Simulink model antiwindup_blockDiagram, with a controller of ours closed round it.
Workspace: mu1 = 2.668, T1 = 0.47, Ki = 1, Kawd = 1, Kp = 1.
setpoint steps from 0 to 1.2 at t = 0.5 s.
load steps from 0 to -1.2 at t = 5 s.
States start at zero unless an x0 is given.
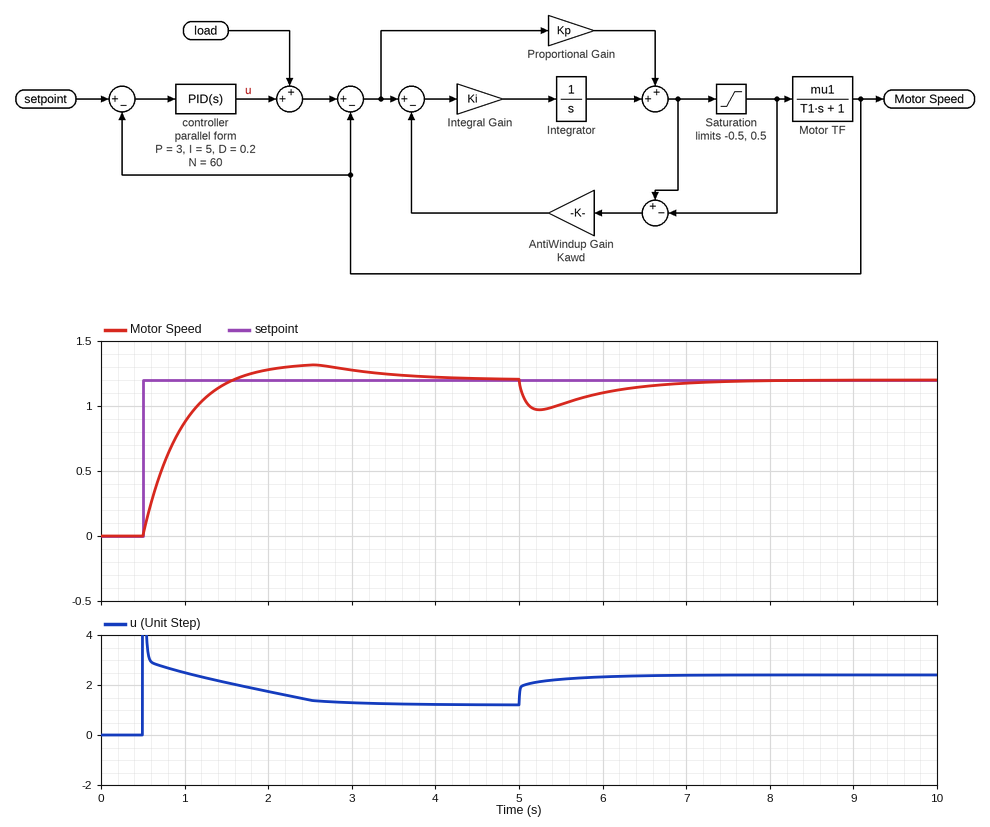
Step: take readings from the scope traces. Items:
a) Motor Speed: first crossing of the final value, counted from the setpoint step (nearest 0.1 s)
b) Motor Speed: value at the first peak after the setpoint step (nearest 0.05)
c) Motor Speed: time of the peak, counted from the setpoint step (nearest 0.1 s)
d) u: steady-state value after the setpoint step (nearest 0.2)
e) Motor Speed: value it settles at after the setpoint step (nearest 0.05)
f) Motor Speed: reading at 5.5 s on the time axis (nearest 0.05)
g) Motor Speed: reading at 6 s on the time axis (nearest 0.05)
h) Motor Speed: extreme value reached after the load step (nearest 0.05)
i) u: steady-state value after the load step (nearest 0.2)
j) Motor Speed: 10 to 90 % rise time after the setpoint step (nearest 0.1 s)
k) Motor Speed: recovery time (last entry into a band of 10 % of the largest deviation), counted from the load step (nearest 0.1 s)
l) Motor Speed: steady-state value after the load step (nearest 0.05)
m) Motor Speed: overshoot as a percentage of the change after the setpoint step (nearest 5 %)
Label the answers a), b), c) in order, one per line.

a) 1.1 s
b) 1.30
c) 2.0 s
d) 1.2
e) 1.20
f) 1.00
g) 1.10
h) 0.95
i) 2.4
j) 0.7 s
k) 2.0 s
l) 1.20
m) 10 %
